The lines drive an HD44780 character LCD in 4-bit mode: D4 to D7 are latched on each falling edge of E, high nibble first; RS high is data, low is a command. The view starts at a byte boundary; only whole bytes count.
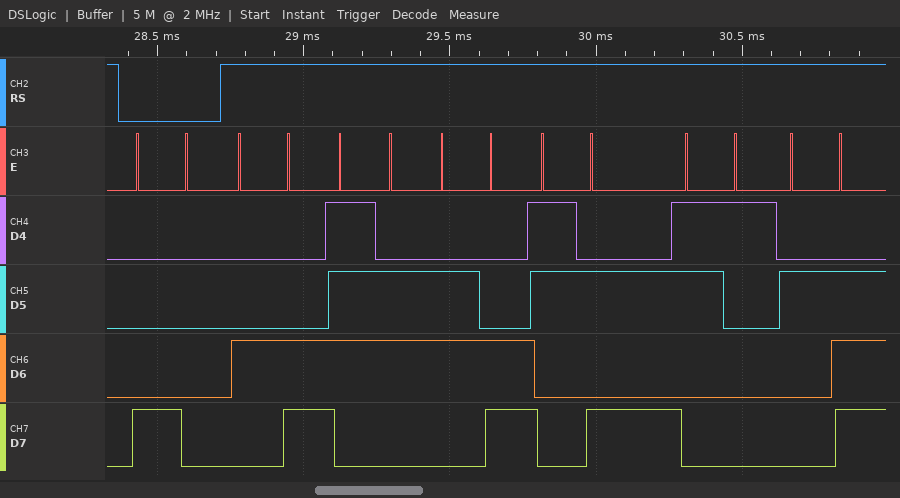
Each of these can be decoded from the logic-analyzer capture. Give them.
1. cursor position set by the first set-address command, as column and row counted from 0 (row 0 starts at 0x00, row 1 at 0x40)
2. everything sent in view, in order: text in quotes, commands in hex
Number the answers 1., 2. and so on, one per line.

1. column 0, row 0
2. 0x80 "Lvl:1."
